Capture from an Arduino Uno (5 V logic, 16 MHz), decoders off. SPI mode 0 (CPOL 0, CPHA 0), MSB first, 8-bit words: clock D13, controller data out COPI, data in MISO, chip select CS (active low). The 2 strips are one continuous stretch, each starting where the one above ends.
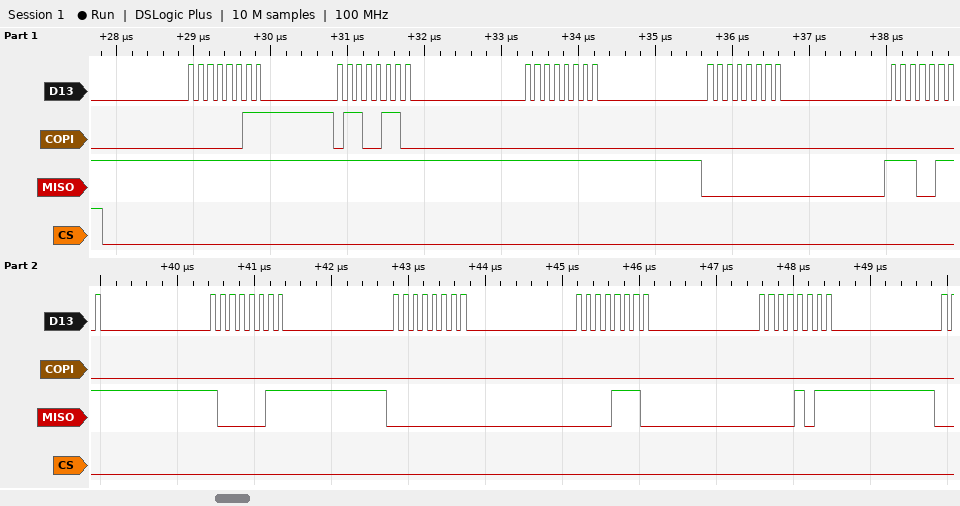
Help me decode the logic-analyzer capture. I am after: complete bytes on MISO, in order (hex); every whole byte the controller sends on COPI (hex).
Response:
FF FF FF 00 E7 83 00 0E 0B
03 66 00 00 00 00 00 00 00
